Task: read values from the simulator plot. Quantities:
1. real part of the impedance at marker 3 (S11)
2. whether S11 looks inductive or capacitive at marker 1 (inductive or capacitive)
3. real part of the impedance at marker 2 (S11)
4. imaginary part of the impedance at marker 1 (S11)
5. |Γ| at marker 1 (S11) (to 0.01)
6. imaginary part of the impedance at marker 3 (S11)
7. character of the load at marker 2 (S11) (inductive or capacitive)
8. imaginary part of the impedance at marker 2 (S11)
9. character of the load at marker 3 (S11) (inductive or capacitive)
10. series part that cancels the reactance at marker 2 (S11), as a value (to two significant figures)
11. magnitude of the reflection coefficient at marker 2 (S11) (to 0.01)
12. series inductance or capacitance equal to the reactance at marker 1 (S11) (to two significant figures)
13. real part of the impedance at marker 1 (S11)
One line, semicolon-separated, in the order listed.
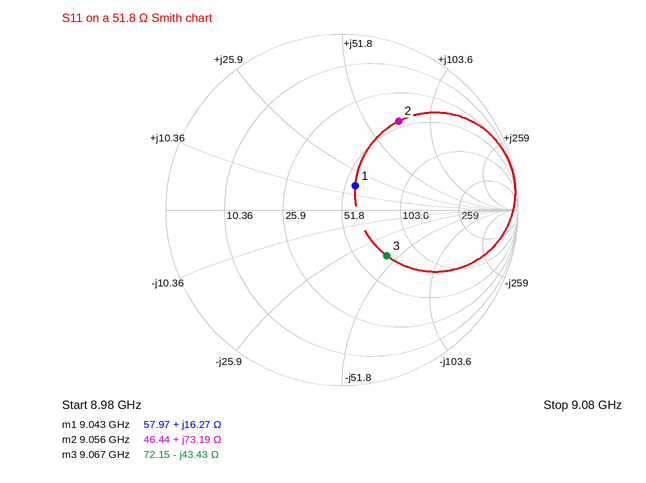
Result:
72.15 Ω; inductive; 46.44 Ω; +16.27 Ω; 0.16; -43.43 Ω; inductive; +73.19 Ω; capacitive; 240 fF; 0.60; 290 pH; 57.97 Ω
